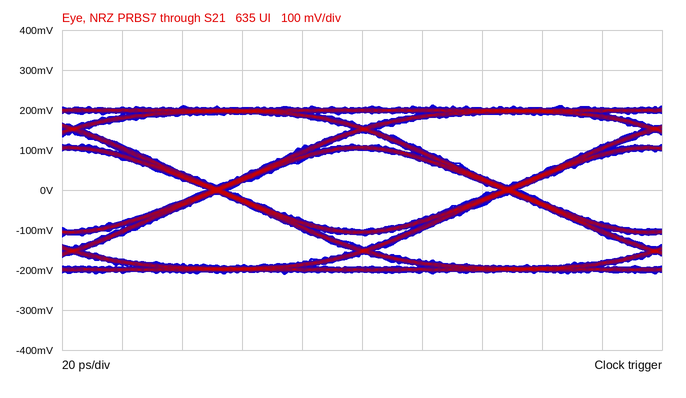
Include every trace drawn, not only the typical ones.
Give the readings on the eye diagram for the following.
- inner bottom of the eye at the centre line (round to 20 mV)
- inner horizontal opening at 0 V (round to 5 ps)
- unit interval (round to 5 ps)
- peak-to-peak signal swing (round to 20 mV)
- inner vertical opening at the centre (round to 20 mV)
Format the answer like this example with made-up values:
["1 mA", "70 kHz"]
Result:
["-100 mV", "90 ps", "95 ps", "420 mV", "200 mV"]
